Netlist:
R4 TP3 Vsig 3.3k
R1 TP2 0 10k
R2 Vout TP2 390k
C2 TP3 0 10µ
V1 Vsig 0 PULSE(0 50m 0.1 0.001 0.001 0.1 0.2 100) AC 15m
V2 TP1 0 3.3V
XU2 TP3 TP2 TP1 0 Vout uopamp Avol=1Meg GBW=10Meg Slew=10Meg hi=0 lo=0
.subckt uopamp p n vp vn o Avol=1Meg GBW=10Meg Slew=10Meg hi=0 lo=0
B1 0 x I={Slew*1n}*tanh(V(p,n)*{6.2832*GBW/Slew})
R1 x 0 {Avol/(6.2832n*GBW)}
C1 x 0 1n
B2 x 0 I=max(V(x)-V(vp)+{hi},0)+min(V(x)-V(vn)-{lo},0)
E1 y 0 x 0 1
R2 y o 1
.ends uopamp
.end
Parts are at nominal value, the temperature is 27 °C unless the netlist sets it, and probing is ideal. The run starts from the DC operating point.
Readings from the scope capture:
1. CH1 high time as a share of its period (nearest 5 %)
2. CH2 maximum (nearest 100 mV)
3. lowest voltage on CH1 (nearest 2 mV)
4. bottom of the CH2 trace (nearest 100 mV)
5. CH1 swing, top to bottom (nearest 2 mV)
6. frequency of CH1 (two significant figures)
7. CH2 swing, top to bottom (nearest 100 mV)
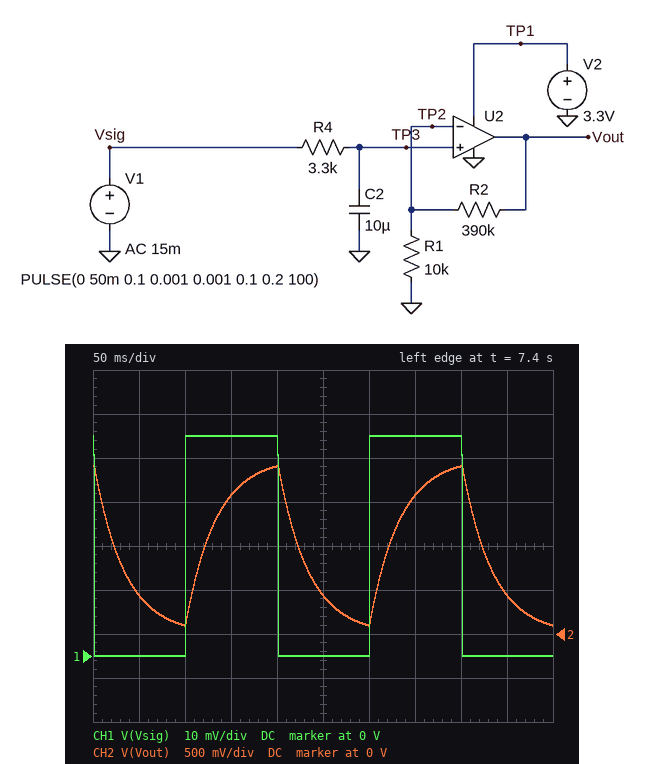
50 %
1.9 V
0 V
100 mV
50 mV
5.0 Hz
1.8 V
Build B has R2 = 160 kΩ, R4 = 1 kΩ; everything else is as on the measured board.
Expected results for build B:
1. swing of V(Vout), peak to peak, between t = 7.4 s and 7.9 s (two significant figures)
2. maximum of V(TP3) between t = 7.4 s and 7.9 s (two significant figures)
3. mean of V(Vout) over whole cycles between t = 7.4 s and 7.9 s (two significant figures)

850 mV
50 mV
430 mV
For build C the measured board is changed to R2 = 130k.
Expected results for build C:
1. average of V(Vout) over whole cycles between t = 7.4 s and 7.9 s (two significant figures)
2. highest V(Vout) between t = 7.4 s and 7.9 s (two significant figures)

350 mV
670 mV
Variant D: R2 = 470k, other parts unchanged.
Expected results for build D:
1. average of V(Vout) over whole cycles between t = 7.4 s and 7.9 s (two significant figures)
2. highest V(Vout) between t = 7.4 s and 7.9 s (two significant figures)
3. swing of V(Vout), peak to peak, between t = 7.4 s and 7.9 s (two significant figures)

1.2 V
2.3 V
2.2 V
